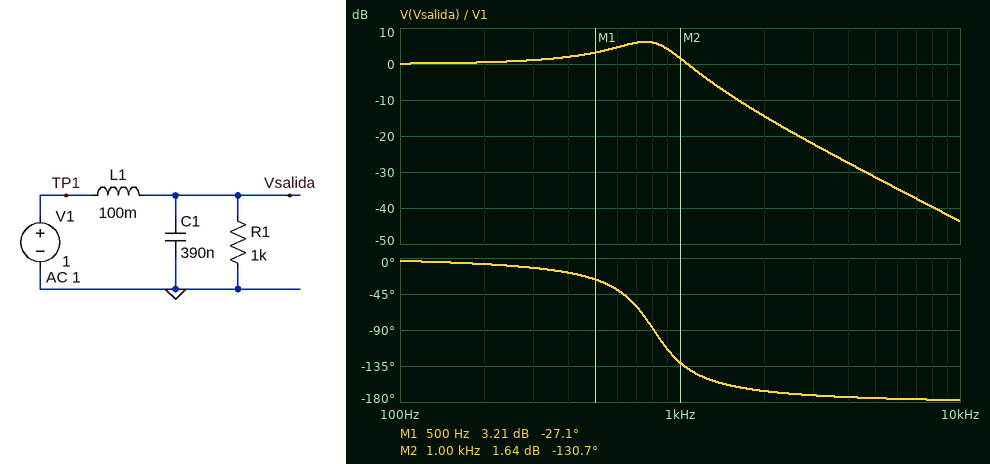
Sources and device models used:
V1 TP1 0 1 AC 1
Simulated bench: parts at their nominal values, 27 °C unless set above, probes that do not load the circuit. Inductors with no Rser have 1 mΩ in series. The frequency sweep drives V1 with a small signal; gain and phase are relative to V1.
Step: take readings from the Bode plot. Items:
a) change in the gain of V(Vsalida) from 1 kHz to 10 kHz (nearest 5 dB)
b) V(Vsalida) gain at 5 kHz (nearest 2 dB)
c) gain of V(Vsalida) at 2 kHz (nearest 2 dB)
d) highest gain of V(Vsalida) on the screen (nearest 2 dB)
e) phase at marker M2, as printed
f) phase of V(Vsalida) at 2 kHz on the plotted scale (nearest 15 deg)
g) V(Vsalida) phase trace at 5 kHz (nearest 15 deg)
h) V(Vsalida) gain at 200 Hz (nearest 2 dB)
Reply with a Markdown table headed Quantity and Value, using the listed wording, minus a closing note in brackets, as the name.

| Quantity | Value |
|---|---|
| change in the gain of V(Vsalida) from 1 kHz to 10 kHz | -45 dB |
| V(Vsalida) gain at 5 kHz | -32 dB |
| gain of V(Vsalida) at 2 kHz | -14 dB |
| highest gain of V(Vsalida) on the screen | 6 dB |
| phase at marker M2, as printed | -130.7 deg |
| phase of V(Vsalida) at 2 kHz on the plotted scale | -165 deg |
| V(Vsalida) phase trace at 5 kHz | -180 deg |
| V(Vsalida) gain at 200 Hz | 0 dB |
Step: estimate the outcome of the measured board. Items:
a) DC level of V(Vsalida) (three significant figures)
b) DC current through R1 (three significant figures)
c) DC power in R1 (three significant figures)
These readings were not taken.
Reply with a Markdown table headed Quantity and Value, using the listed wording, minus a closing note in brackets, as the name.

| Quantity | Value |
|---|---|
| DC level of V(Vsalida) | 1.00 V |
| DC current through R1 | 1.00 mA |
| DC power in R1 | 1.00 mW |
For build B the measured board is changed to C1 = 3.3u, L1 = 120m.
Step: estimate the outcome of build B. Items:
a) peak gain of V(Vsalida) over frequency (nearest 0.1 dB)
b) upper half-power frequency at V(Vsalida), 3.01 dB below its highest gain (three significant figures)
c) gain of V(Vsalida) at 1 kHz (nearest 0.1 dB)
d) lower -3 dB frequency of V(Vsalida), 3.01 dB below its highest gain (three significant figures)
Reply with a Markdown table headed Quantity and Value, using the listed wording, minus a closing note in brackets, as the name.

| Quantity | Value |
|---|---|
| peak gain of V(Vsalida) over frequency | 14.4 dB |
| upper half-power frequency at V(Vsalida), 3.01 dB below its highest gain | 274 Hz |
| gain of V(Vsalida) at 1 kHz | -23.3 dB |
| lower -3 dB frequency of V(Vsalida), 3.01 dB below its highest gain | 225 Hz |
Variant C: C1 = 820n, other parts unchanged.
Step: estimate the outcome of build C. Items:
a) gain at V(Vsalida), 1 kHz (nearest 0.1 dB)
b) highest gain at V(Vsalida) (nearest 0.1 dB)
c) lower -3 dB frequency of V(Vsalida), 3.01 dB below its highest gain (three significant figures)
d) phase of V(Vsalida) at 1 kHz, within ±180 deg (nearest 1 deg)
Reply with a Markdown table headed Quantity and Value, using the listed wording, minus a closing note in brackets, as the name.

| Quantity | Value |
|---|---|
| gain at V(Vsalida), 1 kHz | -7.3 dB |
| highest gain at V(Vsalida) | 9.3 dB |
| lower -3 dB frequency of V(Vsalida), 3.01 dB below its highest gain | 429 Hz |
| phase of V(Vsalida) at 1 kHz, within ±180 deg | -164 deg |
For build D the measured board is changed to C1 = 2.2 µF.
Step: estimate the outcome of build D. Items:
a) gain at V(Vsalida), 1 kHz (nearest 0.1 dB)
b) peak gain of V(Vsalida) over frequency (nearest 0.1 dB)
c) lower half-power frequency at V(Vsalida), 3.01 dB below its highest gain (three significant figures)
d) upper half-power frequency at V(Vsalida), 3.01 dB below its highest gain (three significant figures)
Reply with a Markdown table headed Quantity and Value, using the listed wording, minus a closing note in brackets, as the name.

| Quantity | Value |
|---|---|
| gain at V(Vsalida), 1 kHz | -17.7 dB |
| peak gain of V(Vsalida) over frequency | 13.5 dB |
| lower half-power frequency at V(Vsalida), 3.01 dB below its highest gain | 297 Hz |
| upper half-power frequency at V(Vsalida), 3.01 dB below its highest gain | 370 Hz |
